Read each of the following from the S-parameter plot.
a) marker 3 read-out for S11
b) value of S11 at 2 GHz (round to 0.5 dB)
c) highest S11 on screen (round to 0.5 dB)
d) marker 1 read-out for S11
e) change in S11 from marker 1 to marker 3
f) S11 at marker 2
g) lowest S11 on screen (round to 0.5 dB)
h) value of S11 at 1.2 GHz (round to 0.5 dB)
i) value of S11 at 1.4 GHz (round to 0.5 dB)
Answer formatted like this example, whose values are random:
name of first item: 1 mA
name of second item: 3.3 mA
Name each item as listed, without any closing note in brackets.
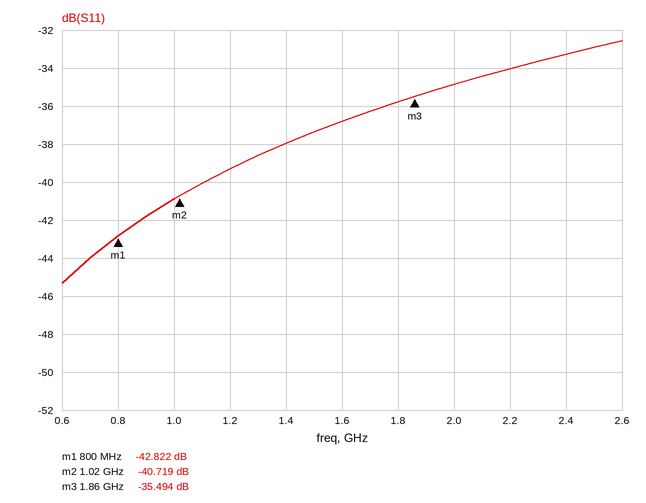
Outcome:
marker 3 read-out for S11: -35.494 dB
value of S11 at 2 GHz: -35.0 dB
highest S11 on screen: -32.5 dB
marker 1 read-out for S11: -42.822 dB
change in S11 from marker 1 to marker 3: 7.328 dB
S11 at marker 2: -40.719 dB
lowest S11 on screen: -45.5 dB
value of S11 at 1.2 GHz: -39.5 dB
value of S11 at 1.4 GHz: -38.0 dB
